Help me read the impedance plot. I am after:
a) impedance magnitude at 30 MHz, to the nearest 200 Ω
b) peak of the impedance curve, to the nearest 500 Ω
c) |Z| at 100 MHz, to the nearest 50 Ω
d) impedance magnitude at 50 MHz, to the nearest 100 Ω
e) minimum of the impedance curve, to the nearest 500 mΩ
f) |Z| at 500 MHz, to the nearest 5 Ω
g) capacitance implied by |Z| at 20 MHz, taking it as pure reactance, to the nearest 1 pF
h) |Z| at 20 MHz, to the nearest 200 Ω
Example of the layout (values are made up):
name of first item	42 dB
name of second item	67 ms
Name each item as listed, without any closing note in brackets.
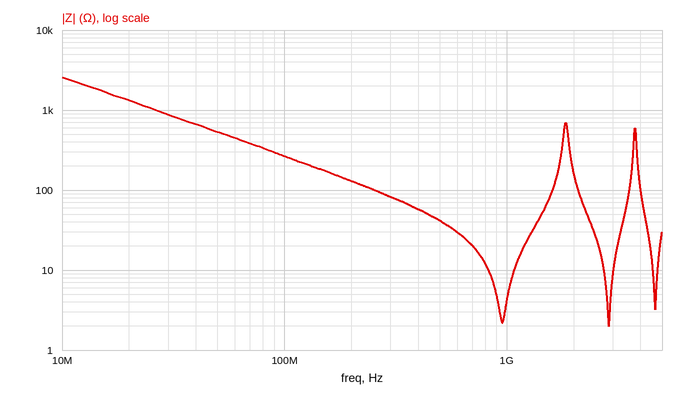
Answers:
impedance magnitude at 30 MHz, to the nearest 200 Ω	800 Ω
peak of the impedance curve, to the nearest 500 Ω	2.5 kΩ
|Z| at 100 MHz, to the nearest 50 Ω	250 Ω
impedance magnitude at 50 MHz, to the nearest 100 Ω	500 Ω
minimum of the impedance curve, to the nearest 500 mΩ	2.0 Ω
|Z| at 500 MHz, to the nearest 5 Ω	40 Ω
capacitance implied by |Z| at 20 MHz, taking it as pure reactance, to the nearest 1 pF	6 pF
|Z| at 20 MHz, to the nearest 200 Ω	1.4 kΩ
